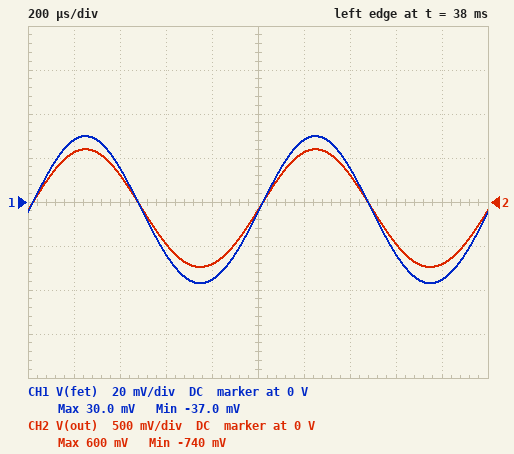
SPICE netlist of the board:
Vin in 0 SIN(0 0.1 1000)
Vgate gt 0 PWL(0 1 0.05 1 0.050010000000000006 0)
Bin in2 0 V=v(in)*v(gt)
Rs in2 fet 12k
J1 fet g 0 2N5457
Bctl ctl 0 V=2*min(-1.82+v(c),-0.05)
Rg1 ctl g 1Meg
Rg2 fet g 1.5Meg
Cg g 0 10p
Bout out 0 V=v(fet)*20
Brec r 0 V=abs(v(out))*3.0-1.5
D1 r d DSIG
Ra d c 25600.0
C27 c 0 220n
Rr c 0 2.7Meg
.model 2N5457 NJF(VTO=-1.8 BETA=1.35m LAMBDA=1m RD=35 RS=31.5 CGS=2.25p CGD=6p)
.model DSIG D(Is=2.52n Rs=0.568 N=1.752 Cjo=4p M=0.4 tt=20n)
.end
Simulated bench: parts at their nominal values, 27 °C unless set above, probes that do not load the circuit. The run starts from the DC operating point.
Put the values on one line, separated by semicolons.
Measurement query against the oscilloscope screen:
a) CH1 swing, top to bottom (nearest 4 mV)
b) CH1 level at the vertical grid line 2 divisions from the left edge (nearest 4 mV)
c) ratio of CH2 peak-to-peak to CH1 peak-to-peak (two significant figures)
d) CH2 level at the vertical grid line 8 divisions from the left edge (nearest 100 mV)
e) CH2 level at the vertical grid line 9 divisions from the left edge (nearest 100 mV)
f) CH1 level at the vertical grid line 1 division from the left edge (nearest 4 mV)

68 mV; 16 mV; 20; -500 mV; -700 mV; 28 mV
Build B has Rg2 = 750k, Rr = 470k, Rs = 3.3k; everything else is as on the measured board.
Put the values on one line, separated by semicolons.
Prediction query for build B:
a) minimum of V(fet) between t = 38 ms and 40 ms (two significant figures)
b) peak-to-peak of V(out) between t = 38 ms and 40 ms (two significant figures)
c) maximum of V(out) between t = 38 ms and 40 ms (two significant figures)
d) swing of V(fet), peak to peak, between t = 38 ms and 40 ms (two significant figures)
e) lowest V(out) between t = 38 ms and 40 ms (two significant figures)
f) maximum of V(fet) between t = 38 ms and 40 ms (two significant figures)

-32 mV; 1.2 V; 550 mV; 59 mV; -630 mV; 27 mV
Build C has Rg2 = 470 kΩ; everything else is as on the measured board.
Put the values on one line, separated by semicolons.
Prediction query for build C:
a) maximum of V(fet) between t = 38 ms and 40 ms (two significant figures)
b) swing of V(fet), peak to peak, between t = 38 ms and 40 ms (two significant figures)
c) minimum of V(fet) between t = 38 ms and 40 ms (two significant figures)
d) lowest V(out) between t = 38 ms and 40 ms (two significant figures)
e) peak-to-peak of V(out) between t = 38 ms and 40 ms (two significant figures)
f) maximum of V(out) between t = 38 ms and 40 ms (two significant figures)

3.6 mV; 10 mV; -6.7 mV; -130 mV; 210 mV; 72 mV
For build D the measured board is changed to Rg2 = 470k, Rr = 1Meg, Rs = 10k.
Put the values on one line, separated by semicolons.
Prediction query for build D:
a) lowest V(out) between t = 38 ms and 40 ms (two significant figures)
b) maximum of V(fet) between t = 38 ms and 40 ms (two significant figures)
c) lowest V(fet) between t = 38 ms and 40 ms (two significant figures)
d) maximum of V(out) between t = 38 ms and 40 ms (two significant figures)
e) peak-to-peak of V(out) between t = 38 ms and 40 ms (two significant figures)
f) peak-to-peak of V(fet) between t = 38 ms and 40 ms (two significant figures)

-150 mV; 4.6 mV; -7.6 mV; 92 mV; 240 mV; 12 mV
